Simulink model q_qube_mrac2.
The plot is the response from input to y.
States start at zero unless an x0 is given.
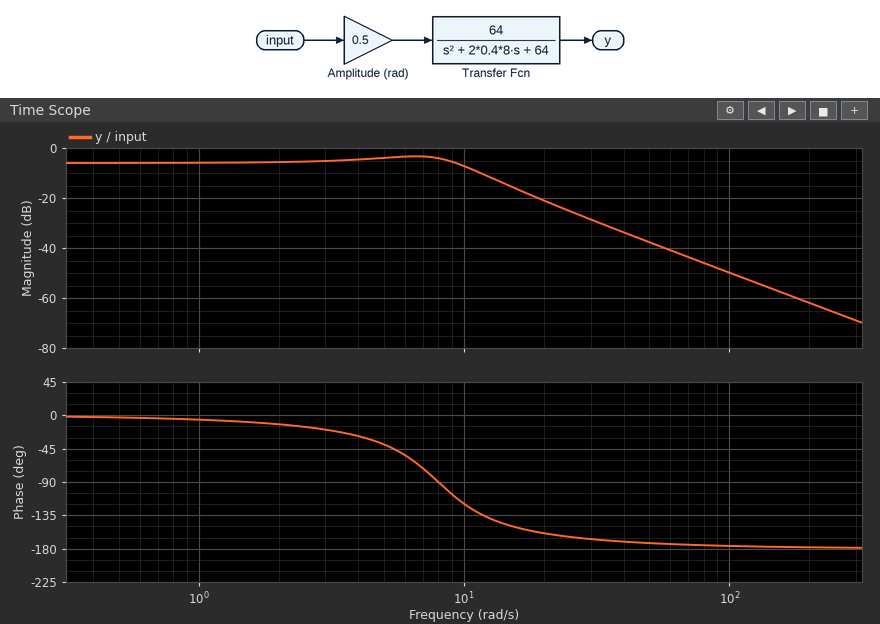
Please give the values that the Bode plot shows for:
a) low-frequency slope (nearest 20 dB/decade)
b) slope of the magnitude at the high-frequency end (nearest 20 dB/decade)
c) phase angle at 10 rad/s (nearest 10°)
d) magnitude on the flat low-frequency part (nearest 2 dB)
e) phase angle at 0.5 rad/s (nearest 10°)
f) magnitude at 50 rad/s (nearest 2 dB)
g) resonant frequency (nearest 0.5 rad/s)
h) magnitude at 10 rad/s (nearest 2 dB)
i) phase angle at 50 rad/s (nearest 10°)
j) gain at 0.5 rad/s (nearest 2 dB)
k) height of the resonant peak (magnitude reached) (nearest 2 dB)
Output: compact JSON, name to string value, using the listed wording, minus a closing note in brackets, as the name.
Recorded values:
{"low-frequency slope": "0 dB/decade", "slope of the magnitude at the high-frequency end": "-40 dB/decade", "phase angle at 10 rad/s": "-120°", "magnitude on the flat low-frequency part": "-6 dB", "phase angle at 0.5 rad/s": "0°", "magnitude at 50 rad/s": "-38 dB", "resonant frequency": "6.5 rad/s", "magnitude at 10 rad/s": "-8 dB", "phase angle at 50 rad/s": "-170°", "gain at 0.5 rad/s": "-6 dB", "height of the resonant peak (magnitude reached)": "-4 dB"}
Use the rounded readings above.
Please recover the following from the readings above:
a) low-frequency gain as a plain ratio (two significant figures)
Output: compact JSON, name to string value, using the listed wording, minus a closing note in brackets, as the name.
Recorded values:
{"low-frequency gain as a plain ratio": "0.50"}
